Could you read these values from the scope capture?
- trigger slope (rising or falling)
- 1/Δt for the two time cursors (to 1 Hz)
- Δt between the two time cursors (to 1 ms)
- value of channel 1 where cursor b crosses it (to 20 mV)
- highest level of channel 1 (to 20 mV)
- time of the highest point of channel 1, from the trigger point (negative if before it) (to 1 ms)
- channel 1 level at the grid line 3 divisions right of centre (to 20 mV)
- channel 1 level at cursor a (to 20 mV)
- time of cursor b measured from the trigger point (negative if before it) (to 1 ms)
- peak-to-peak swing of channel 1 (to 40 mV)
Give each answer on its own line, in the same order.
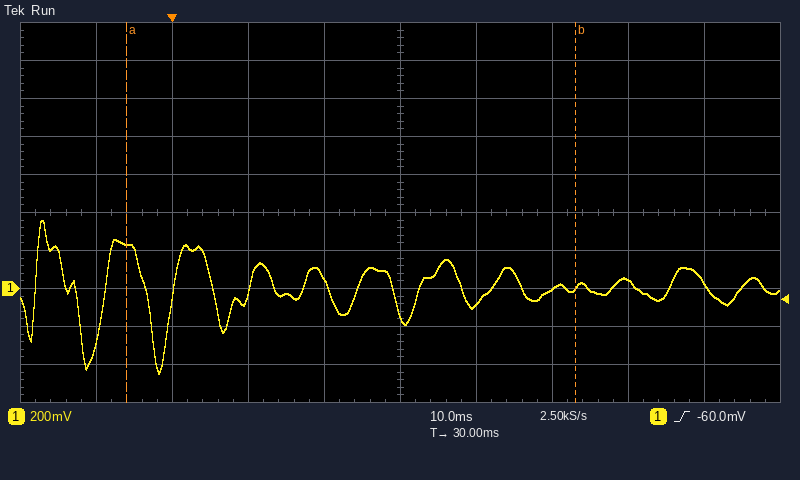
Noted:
rising
17 Hz
59 ms
0 mV
360 mV
-17 ms
40 mV
240 mV
+53 ms
800 mV
